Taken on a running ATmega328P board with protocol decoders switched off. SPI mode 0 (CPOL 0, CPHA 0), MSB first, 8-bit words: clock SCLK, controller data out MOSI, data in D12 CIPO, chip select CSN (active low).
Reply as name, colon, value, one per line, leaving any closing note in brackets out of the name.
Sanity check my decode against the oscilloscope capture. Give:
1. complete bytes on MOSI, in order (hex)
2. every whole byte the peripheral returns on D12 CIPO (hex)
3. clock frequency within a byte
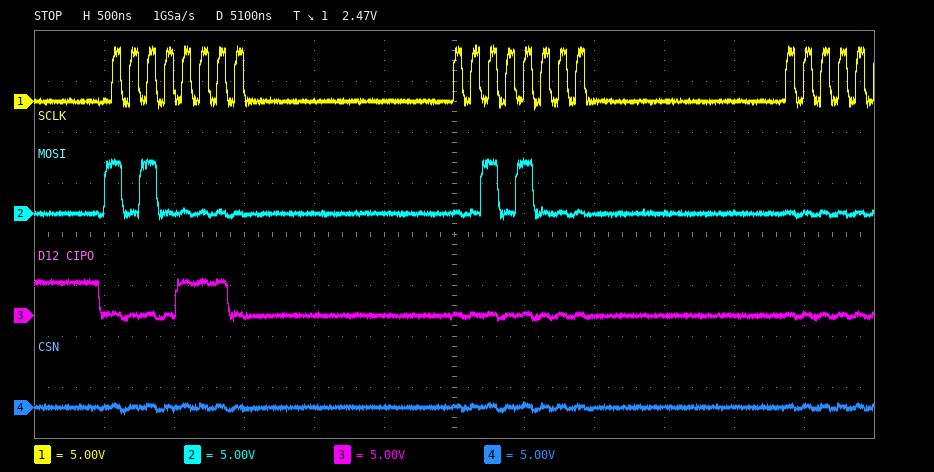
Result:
complete bytes on MOSI, in order: A0 28
every whole byte the peripheral returns on D12 CIPO: 0E 00
clock frequency within a byte: 8 MHz
